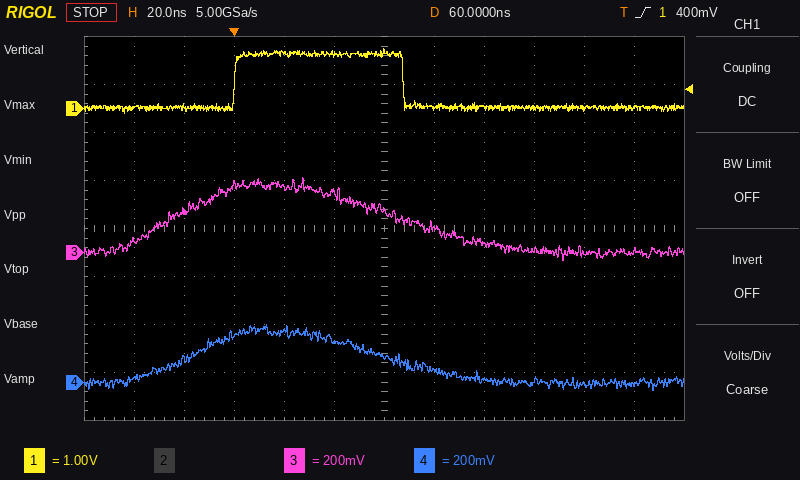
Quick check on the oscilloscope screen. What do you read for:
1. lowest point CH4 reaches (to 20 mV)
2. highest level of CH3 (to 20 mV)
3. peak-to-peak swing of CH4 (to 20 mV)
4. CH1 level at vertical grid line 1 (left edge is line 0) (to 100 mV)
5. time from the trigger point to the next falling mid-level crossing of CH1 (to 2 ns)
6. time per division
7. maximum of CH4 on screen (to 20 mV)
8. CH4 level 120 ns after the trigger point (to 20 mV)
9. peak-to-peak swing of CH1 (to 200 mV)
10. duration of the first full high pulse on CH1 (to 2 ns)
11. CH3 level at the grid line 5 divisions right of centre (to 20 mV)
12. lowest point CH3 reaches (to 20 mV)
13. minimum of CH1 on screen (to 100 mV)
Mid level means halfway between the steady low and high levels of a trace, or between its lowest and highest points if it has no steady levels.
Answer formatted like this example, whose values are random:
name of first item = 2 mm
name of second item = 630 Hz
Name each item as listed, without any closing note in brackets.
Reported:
lowest point CH4 reaches = -40 mV
highest level of CH3 = 320 mV
peak-to-peak swing of CH4 = 280 mV
CH1 level at vertical grid line 1 (left edge is line 0) = 0.0 V
time from the trigger point to the next falling mid-level crossing of CH1 = 68 ns
time per division = 20 ns
maximum of CH4 on screen = 240 mV
CH4 level 120 ns after the trigger point = 0 mV
peak-to-peak swing of CH1 = 1.4 V
duration of the first full high pulse on CH1 = 68 ns
CH3 level at the grid line 5 divisions right of centre = 0 mV
lowest point CH3 reaches = -40 mV
minimum of CH1 on screen = -100 mV
